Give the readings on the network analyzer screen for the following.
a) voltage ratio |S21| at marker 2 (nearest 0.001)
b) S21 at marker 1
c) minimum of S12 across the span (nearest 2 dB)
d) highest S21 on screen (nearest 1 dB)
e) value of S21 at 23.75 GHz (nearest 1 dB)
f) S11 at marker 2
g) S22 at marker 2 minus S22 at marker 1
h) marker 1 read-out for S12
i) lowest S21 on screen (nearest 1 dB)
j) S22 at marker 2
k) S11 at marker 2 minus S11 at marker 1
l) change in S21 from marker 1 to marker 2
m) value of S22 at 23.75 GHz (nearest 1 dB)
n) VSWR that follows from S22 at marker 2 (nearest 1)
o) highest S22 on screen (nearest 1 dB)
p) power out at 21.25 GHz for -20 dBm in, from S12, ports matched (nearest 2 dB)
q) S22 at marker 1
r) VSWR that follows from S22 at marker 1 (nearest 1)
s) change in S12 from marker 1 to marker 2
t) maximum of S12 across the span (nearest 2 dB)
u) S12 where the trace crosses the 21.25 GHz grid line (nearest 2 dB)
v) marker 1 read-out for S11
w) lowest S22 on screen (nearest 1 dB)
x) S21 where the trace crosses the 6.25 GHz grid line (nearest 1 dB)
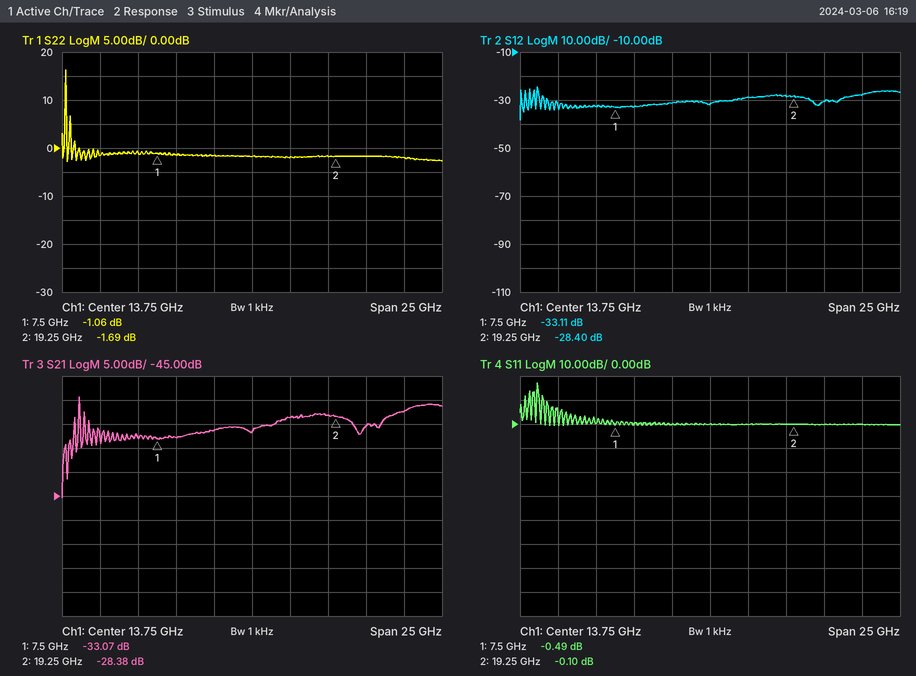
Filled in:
0.038
-33.07 dB
-38 dB
-24 dB
-27 dB
-0.10 dB
-0.63 dB
-33.11 dB
-45 dB
-1.69 dB
0.39 dB
4.69 dB
-2 dB
10
16 dB
-50 dBm
-1.06 dB
16
4.71 dB
-24 dB
-30 dB
-0.49 dB
-3 dB
-33 dB
